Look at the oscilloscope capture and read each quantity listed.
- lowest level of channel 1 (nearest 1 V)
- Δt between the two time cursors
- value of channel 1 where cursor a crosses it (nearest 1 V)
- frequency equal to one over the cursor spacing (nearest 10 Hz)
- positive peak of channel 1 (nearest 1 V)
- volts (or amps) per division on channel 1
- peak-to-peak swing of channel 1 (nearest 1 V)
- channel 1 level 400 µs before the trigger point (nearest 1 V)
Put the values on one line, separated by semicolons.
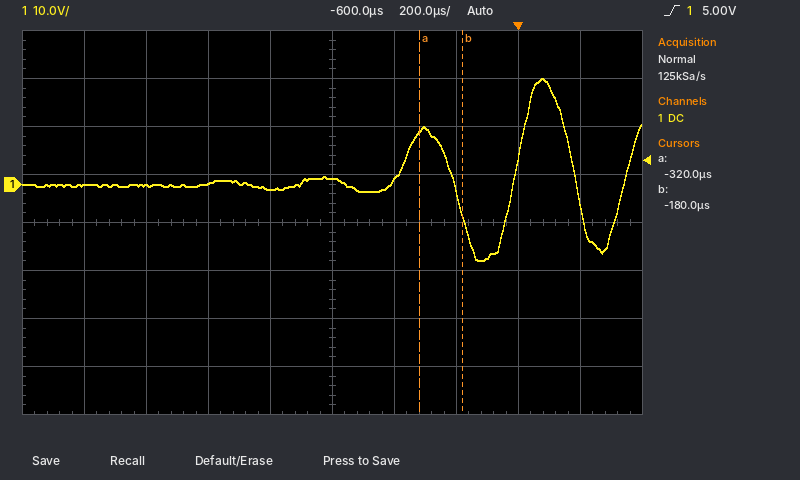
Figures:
-16 V; 140 µs; 11 V; 7.14 kHz; 22 V; 10 V; 38 V; 1 V
